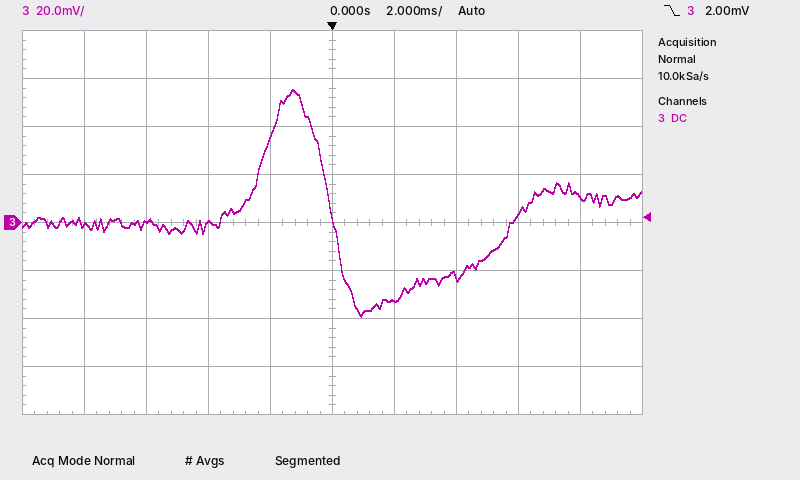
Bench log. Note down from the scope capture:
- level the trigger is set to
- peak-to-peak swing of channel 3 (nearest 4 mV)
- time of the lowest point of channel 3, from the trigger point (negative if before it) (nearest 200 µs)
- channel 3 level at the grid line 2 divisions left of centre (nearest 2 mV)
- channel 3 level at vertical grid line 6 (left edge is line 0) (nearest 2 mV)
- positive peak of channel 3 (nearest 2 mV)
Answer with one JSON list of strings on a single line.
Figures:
["2.00 mV", "96 mV", "+1.0 ms", "0 mV", "-32 mV", "56 mV"]
